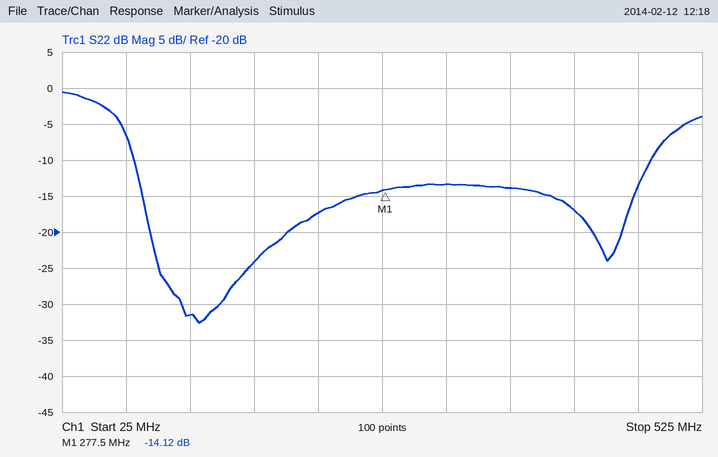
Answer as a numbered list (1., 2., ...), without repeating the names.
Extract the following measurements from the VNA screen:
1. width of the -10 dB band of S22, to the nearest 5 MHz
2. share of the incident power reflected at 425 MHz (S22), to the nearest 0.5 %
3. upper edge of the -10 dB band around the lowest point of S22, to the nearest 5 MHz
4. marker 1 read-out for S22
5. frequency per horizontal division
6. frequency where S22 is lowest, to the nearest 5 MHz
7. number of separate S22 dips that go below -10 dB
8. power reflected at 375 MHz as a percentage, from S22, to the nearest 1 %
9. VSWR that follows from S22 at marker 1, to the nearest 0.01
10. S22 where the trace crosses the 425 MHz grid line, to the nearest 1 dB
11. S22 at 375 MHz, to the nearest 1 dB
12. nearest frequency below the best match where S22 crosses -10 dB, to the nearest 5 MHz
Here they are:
1. 405 MHz
2. 2.0 %
3. 485 MHz
4. -14.12 dB
5. 50 MHz
6. 130 MHz
7. 2
8. 4 %
9. 1.49
10. -17 dB
11. -14 dB
12. 80 MHz
